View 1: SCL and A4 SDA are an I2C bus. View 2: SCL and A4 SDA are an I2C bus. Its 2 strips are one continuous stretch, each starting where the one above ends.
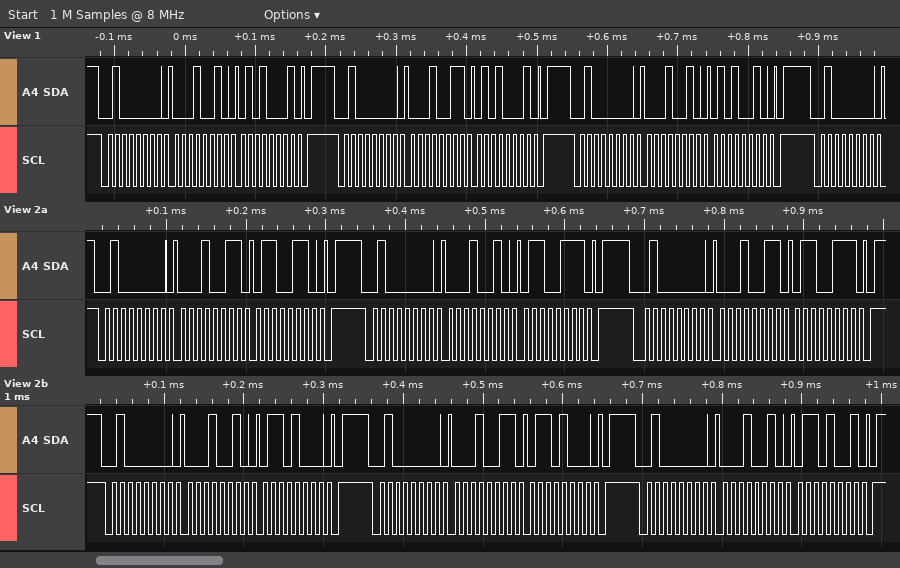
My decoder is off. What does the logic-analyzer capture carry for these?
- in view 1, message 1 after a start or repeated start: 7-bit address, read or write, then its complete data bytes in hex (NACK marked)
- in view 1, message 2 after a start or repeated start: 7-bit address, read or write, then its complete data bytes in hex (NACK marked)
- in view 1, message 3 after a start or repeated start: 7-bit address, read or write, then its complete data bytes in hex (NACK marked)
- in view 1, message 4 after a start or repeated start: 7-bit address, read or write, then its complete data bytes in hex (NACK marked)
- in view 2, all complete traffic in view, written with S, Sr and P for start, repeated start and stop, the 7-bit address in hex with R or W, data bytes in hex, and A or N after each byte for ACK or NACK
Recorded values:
0x20 write: 12 51
0x20 write: 13 51
0x20 write: 12 52
0x20 write
S 20W A 13 A 66 A P S 20W A 12 A 67 A P S 20W A 13 A 67 A P S 20W A 12 A 68 A P S 20W A 13 A 68 A P S 20W A 12 A 69 A P
